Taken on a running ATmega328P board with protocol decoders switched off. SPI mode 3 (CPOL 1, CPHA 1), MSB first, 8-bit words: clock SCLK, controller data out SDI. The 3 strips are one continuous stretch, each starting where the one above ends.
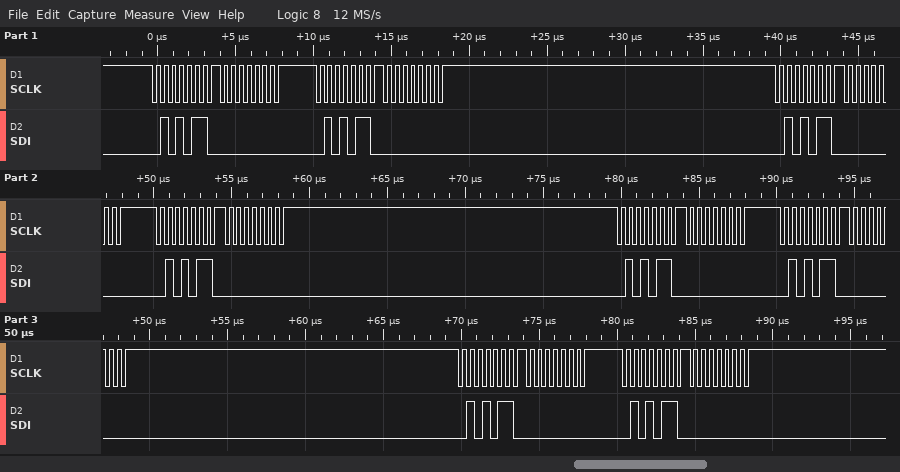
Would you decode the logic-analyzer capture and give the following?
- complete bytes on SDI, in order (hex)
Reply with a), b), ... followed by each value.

a) 56 00 56 00 56 00 56 00 56 00 56 00 56 00 56 00
